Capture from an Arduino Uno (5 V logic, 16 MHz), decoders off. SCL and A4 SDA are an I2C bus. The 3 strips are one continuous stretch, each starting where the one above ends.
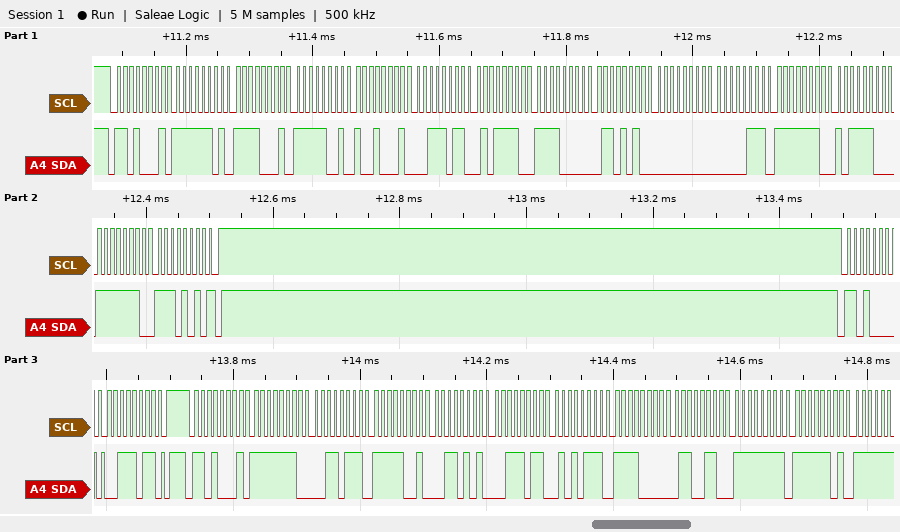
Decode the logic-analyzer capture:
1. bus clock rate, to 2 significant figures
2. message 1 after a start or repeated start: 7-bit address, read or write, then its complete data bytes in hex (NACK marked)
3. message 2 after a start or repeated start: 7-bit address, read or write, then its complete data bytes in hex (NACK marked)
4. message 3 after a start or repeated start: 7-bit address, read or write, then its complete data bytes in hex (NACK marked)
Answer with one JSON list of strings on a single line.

["100 kHz", "0x68 read: FD F1 F9 91 3B 5E F0 6A 00 07 FE BC FE EA NACK", "0x68 write: 3B", "0x68 read: FE 37 F9 35 3B 57 F0 66 FF FD"]
